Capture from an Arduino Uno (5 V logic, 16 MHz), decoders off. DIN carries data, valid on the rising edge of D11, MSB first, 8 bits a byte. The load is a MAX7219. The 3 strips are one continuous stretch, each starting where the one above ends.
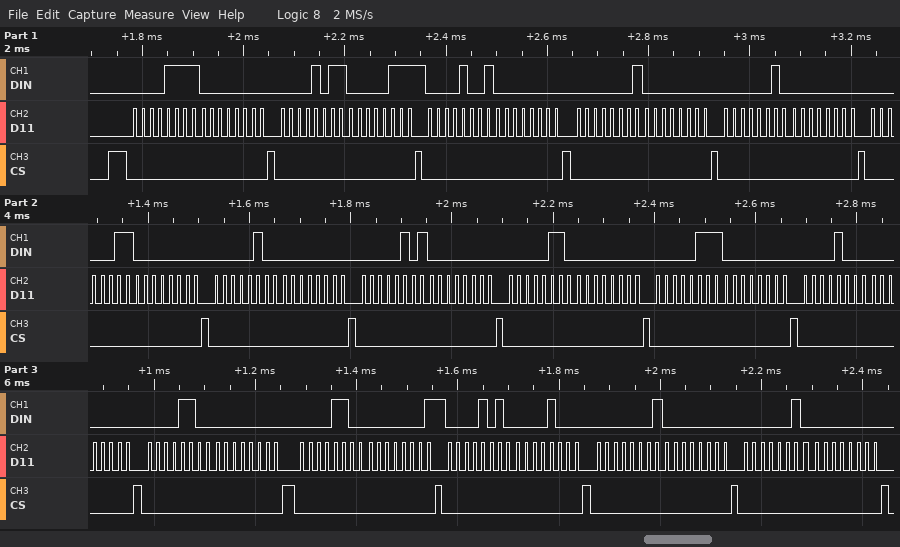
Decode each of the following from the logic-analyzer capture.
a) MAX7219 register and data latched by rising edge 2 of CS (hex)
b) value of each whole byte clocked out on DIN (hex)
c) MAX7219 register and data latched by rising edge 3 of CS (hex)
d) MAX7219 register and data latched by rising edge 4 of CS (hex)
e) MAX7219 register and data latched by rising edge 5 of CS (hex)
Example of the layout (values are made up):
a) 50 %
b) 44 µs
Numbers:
a) register 0xF, data 0x00
b) 0x0F 0x00 0x0B 0x07 0x09 0x00 0x01 0x00 0x02 0x00 0x03 0x00 0x04 0x00 0x05 0x00 0x06 0x00 0x07 0x00 0x08 0x00 0x0C 0x00 0x0C 0x01 0x0A 0x08 0x01 0x00 0x02 0x00
c) register 0xB, data 0x07
d) register 0x9, data 0x00
e) register 0x1, data 0x00
